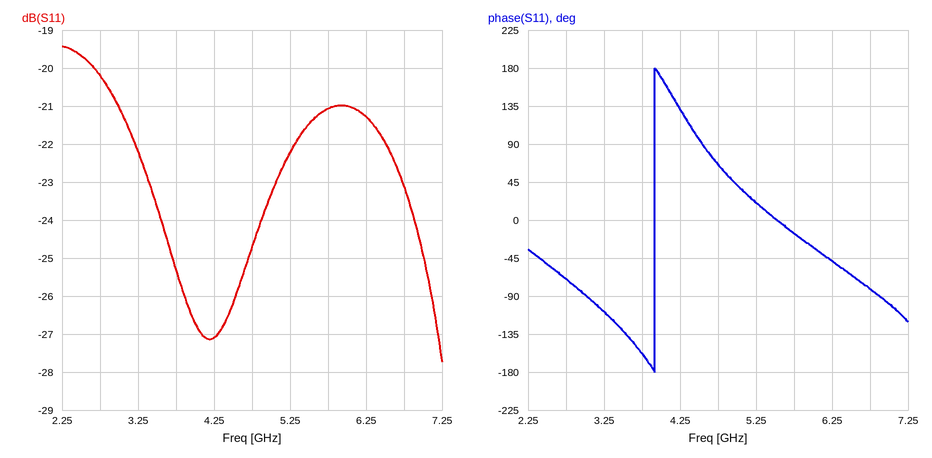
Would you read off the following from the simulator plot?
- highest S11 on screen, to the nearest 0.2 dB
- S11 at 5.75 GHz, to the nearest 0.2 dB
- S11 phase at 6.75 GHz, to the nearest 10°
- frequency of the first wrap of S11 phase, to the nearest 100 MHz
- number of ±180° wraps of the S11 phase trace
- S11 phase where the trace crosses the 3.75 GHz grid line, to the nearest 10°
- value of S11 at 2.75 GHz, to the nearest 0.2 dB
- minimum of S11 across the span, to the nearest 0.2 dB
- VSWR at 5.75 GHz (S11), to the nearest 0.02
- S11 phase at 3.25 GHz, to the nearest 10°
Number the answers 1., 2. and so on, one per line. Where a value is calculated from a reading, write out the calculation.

1. -19.4 dB
2. -21.0 dB
3. -80°
4. 3.9 GHz
5. 1
6. -160°
7. -20.2 dB
8. -27.8 dB
9. |Γ| = 10^(-21/20) = 0.0891; VSWR = (1 + 0.0891)/(1 − 0.0891) ≈ 1.20
10. -110°
